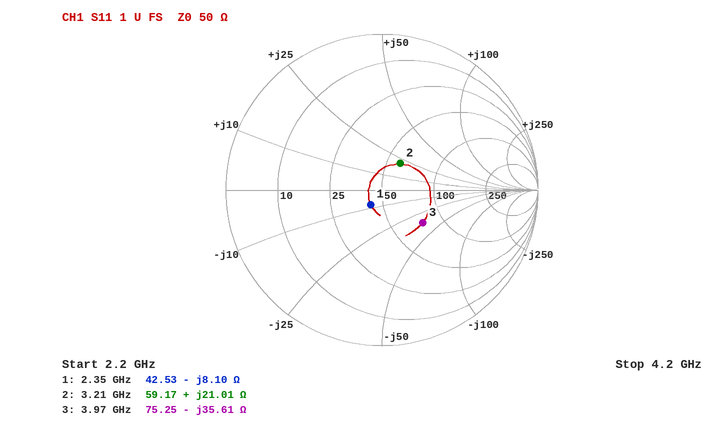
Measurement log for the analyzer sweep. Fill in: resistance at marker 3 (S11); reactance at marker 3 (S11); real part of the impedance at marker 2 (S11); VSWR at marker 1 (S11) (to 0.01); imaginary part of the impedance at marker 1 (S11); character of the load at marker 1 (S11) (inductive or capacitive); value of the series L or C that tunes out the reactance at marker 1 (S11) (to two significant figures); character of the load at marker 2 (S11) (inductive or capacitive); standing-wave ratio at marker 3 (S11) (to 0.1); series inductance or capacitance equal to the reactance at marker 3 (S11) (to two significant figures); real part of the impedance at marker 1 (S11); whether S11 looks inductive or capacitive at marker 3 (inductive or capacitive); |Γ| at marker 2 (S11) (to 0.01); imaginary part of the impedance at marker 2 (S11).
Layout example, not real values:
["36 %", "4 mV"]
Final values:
["75.25 Ω", "-35.61 Ω", "59.17 Ω", "1.27", "-8.10 Ω", "capacitive", "550 pH", "inductive", "2.0", "1.1 pF", "42.53 Ω", "capacitive", "0.21", "+21.01 Ω"]
